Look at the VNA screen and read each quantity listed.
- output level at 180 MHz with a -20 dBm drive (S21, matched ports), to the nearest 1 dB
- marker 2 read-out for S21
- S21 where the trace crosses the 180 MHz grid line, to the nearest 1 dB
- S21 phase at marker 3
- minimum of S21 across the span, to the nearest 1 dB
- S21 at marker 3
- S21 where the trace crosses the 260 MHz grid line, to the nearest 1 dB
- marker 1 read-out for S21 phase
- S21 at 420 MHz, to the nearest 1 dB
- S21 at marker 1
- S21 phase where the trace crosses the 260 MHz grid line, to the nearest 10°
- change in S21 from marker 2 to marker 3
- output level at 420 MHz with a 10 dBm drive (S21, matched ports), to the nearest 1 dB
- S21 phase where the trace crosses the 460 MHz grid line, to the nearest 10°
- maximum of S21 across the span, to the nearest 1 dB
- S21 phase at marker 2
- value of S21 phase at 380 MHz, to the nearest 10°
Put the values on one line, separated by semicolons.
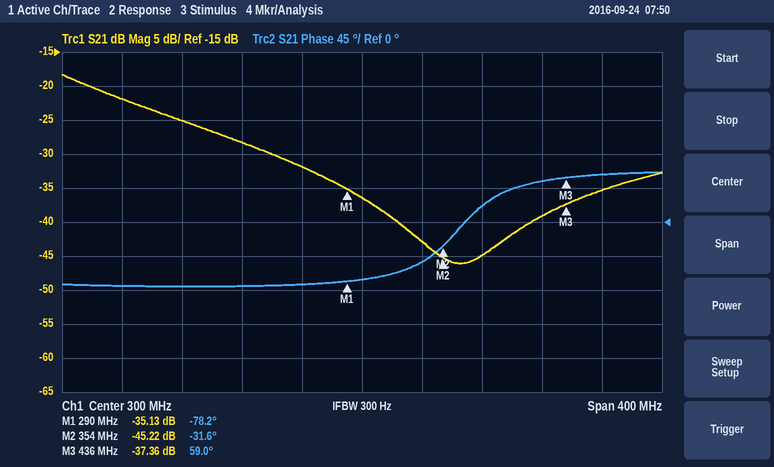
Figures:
-45 dBm; -45.22 dB; -25 dB; 59.0°; -46 dB; -37.36 dB; -32 dB; -78.2°; -39 dB; -35.13 dB; -80°; 7.86 dB; -29 dBm; 60°; -18 dB; -31.6°; 20°
